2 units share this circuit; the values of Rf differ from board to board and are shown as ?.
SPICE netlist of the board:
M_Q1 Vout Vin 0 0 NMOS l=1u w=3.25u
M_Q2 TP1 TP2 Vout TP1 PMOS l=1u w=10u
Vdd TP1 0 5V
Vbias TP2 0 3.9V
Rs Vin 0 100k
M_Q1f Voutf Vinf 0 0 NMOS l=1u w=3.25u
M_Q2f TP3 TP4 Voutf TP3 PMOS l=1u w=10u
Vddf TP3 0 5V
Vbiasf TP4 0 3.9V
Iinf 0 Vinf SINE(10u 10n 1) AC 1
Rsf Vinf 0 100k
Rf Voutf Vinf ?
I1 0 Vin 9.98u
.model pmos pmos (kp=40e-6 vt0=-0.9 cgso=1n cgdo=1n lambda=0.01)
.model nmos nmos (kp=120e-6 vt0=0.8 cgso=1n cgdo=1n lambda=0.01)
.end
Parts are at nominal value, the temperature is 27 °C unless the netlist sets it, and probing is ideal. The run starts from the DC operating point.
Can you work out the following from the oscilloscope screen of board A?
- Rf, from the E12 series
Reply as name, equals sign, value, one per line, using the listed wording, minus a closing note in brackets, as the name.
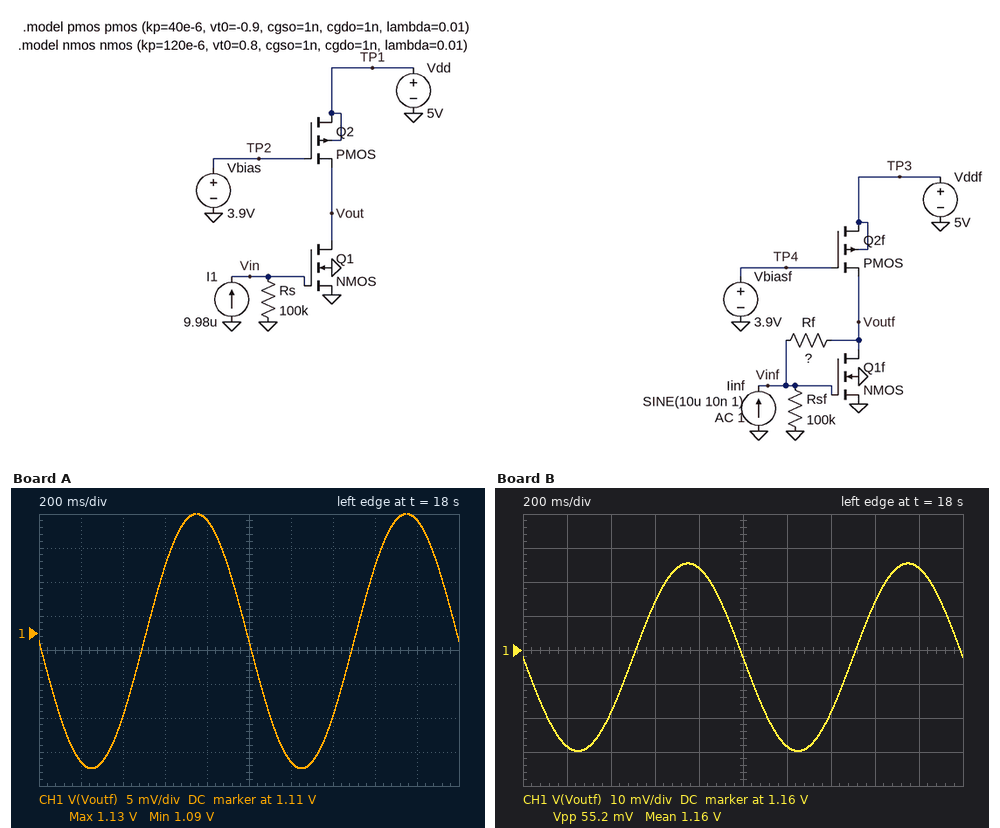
Rf, from the E12 series = 2.2 MΩ
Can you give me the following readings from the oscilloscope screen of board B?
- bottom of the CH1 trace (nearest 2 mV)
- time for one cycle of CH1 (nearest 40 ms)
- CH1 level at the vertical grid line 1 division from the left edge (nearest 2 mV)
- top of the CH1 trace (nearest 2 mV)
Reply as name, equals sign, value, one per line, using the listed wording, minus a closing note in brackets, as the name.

bottom of the CH1 trace = 1.130 V
time for one cycle of CH1 = 1.00 s
CH1 level at the vertical grid line 1 division from the left edge = 1.132 V
top of the CH1 trace = 1.186 V
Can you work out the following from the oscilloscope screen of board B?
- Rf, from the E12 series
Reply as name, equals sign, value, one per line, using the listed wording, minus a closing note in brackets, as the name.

Rf, from the E12 series = 3.3 MΩ
